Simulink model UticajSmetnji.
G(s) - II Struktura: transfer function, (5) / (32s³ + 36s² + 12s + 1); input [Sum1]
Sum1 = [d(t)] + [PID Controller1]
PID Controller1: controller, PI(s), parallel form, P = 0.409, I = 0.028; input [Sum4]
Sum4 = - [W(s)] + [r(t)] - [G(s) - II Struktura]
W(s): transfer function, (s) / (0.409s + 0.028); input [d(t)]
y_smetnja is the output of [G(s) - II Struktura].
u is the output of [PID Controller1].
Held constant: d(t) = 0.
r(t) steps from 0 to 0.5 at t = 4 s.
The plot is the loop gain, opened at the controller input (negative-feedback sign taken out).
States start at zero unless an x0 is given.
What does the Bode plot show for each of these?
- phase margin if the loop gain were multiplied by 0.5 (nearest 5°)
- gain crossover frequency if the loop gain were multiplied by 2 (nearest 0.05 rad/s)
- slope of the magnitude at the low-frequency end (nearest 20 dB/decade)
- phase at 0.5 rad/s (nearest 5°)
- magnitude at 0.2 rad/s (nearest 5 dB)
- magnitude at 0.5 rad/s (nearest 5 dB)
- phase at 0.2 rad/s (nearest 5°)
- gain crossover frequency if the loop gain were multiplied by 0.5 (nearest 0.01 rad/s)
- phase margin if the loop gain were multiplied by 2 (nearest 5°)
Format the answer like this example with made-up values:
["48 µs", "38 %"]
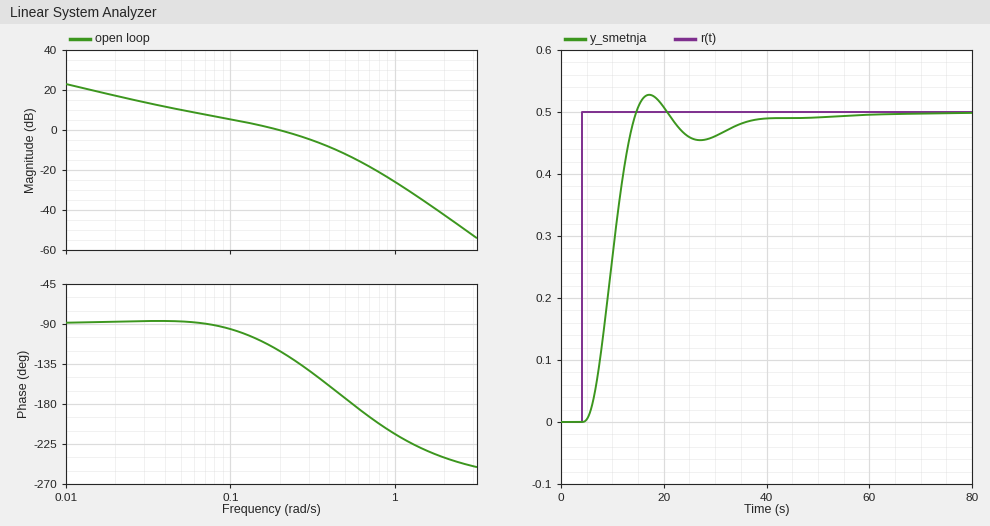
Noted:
["85°", "0.35 rad/s", "-20 dB/decade", "-175°", "0 dB", "-10 dB", "-120°", "0.09 rad/s", "30°"]
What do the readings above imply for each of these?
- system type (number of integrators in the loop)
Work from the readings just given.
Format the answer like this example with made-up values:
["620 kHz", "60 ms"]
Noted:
["1"]
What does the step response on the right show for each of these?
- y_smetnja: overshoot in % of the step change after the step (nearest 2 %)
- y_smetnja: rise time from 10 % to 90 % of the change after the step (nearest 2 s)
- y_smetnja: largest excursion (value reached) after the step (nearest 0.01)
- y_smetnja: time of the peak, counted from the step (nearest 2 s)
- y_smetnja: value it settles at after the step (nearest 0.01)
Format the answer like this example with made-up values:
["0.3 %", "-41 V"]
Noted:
["6 %", "6 s", "0.53", "14 s", "0.50"]
